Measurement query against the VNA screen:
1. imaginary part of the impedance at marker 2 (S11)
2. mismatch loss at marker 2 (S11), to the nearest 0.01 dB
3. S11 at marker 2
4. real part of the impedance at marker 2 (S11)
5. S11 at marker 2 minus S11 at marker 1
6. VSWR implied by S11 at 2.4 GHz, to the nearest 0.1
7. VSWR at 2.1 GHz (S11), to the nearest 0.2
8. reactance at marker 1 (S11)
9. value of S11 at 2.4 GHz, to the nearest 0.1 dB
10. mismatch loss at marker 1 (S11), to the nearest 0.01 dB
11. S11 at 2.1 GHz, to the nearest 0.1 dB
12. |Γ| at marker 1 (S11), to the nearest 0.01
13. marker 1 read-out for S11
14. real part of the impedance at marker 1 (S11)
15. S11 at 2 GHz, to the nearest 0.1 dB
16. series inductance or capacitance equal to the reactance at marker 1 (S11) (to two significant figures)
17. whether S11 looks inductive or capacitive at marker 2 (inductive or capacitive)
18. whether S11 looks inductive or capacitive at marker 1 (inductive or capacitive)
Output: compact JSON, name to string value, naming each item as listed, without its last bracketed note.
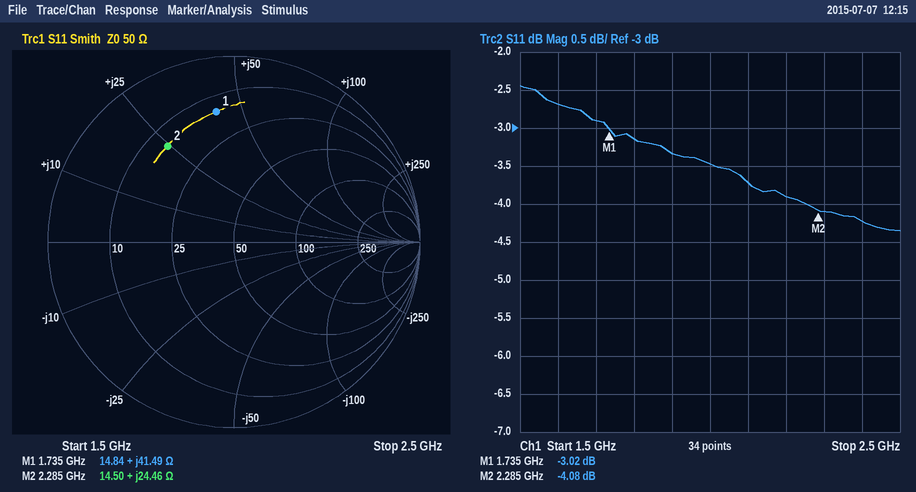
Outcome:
{"imaginary part of the impedance at marker 2": "+24.46 Ω", "mismatch loss at marker 2 (S11), to the nearest 0.01 dB": "2.15 dB", "S11 at marker 2": "-4.08 dB", "real part of the impedance at marker 2": "14.50 Ω", "S11 at marker 2 minus S11 at marker 1": "-1.06 dB", "VSWR implied by S11 at 2.4 GHz, to the nearest 0.1": "4.2", "VSWR at 2.1 GHz (S11), to the nearest 0.2": "4.8", "reactance at marker 1": "+41.49 Ω", "value of S11 at 2.4 GHz, to the nearest 0.1 dB": "-4.2 dB", "mismatch loss at marker 1 (S11), to the nearest 0.01 dB": "3.00 dB", "S11 at 2.1 GHz, to the nearest 0.1 dB": "-3.7 dB", "|Γ| at marker 1 (S11), to the nearest 0.01": "0.71", "marker 1 read-out for S11": "-3.02 dB", "real part of the impedance at marker 1": "14.84 Ω", "S11 at 2 GHz, to the nearest 0.1 dB": "-3.5 dB", "series inductance or capacitance equal to the reactance at marker 1 (S11)": "3.8 nH", "whether S11 looks inductive or capacitive at marker 2": "inductive", "whether S11 looks inductive or capacitive at marker 1": "inductive"}
